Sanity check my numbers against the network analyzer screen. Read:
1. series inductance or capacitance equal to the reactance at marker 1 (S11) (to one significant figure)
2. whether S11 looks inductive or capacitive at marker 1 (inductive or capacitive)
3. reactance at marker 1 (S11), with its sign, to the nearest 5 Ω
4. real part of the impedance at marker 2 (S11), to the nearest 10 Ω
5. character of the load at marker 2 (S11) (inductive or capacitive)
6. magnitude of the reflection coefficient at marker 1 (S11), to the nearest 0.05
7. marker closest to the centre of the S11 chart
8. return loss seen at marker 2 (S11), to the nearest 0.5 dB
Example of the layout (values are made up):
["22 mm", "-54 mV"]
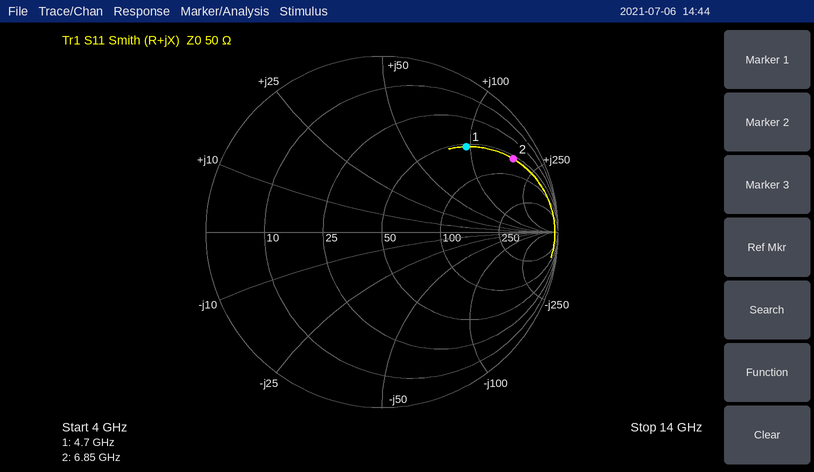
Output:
["3 nH", "inductive", "+95 Ω", "60 Ω", "inductive", "0.70", "marker 1", "1.5 dB"]
